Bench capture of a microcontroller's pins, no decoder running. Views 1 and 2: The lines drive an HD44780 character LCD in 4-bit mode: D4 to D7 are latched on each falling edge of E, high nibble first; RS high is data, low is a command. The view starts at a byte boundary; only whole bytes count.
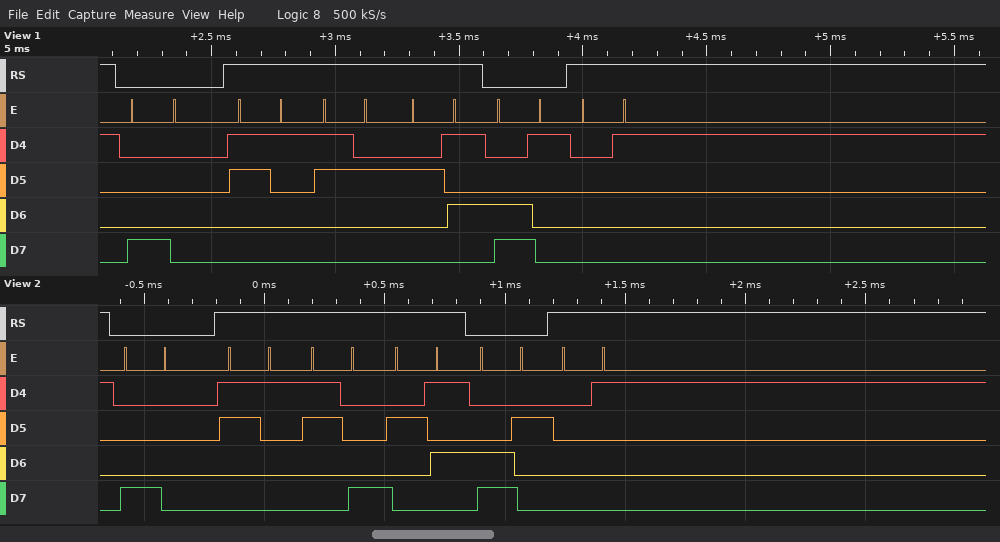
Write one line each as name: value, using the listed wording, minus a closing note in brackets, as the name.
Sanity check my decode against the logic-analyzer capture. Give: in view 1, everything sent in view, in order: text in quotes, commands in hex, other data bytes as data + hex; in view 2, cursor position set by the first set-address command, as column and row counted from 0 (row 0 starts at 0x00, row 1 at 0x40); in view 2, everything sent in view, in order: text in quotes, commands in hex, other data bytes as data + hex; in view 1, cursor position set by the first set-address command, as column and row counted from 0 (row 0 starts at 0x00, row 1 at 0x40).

in view 1, everything sent in view, in order: text in quotes, commands in hex, other data bytes as data + hex: 0x80 "12%" 0xC1 data 01
in view 2, cursor position set by the first set-address command, as column and row counted from 0: column 0, row 0
in view 2, everything sent in view, in order: text in quotes, commands in hex, other data bytes as data + hex: 0x80 "18%" 0xC2 data 01
in view 1, cursor position set by the first set-address command, as column and row counted from 0: column 0, row 0
